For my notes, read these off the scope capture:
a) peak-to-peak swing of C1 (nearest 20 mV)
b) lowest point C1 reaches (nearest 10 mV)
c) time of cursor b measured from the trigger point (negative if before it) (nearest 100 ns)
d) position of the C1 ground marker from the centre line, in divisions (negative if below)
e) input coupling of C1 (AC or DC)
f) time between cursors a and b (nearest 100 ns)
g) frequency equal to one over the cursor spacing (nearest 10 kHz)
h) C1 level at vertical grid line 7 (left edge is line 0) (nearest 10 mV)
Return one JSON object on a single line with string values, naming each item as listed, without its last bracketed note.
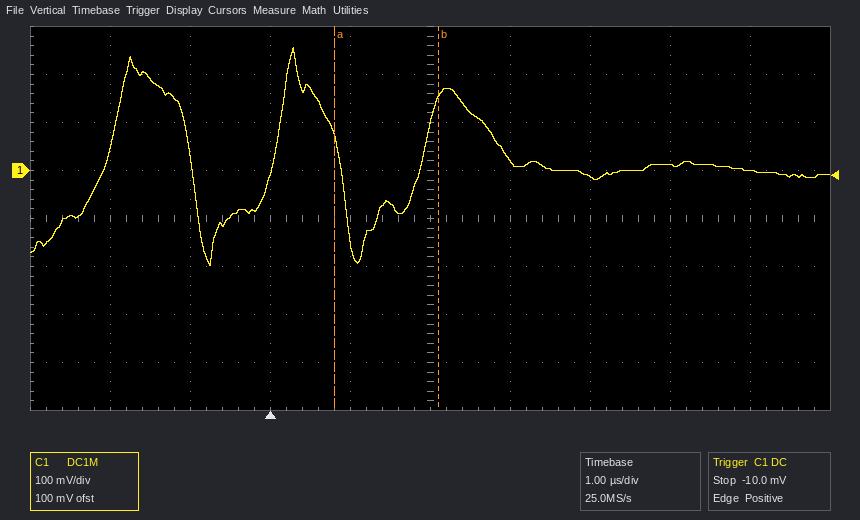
{"peak-to-peak swing of C1": "460 mV", "lowest point C1 reaches": "-200 mV", "time of cursor b measured from the trigger point (negative if before it)": "+2.1 µs", "position of the C1 ground marker from the centre line, in divisions": "+1.0 div", "input coupling of C1": "DC", "time between cursors a and b": "1.3 µs", "frequency equal to one over the cursor spacing": "770 kHz", "C1 level at vertical grid line 7 (left edge is line 0)": "-10 mV"}
